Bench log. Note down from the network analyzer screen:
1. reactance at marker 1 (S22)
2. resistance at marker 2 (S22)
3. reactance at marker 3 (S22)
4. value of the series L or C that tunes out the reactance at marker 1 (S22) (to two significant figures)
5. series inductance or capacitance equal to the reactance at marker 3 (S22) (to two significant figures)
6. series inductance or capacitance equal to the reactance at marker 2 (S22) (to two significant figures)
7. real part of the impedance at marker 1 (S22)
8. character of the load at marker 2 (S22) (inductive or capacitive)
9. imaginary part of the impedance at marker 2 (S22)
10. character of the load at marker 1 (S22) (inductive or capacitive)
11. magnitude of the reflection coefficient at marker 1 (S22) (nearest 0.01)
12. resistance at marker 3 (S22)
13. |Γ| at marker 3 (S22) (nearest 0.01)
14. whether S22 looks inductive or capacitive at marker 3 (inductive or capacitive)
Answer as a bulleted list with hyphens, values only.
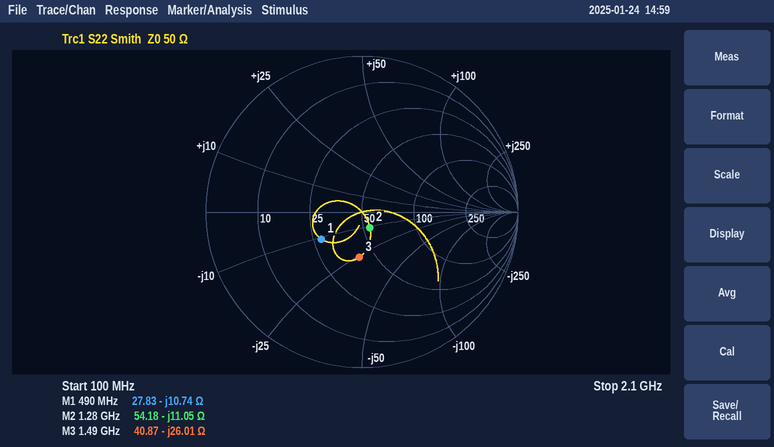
- -10.74 Ω
- 54.18 Ω
- -26.01 Ω
- 3.5 nH
- 4.1 pF
- 11 pF
- 27.83 Ω
- capacitive
- -11.05 Ω
- capacitive
- 0.31
- 40.87 Ω
- 0.29
- capacitive
